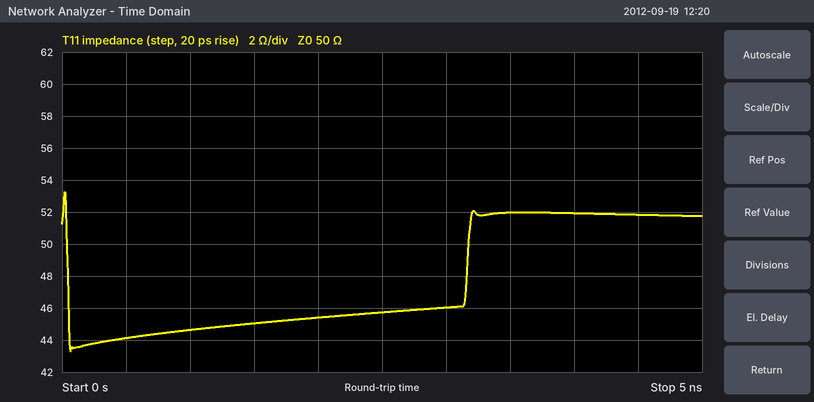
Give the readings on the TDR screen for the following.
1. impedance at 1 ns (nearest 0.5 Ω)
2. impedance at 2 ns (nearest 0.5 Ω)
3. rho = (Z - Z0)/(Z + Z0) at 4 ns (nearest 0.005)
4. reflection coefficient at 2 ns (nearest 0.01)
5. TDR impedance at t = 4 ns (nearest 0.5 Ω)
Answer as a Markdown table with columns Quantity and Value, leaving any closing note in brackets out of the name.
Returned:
| Quantity | Value |
|---|---|
| impedance at 1 ns | 44.5 Ω |
| impedance at 2 ns | 45.5 Ω |
| rho = (Z - Z0)/(Z + Z0) at 4 ns | +0.020 |
| reflection coefficient at 2 ns | -0.05 |
| TDR impedance at t = 4 ns | 52.0 Ω |
